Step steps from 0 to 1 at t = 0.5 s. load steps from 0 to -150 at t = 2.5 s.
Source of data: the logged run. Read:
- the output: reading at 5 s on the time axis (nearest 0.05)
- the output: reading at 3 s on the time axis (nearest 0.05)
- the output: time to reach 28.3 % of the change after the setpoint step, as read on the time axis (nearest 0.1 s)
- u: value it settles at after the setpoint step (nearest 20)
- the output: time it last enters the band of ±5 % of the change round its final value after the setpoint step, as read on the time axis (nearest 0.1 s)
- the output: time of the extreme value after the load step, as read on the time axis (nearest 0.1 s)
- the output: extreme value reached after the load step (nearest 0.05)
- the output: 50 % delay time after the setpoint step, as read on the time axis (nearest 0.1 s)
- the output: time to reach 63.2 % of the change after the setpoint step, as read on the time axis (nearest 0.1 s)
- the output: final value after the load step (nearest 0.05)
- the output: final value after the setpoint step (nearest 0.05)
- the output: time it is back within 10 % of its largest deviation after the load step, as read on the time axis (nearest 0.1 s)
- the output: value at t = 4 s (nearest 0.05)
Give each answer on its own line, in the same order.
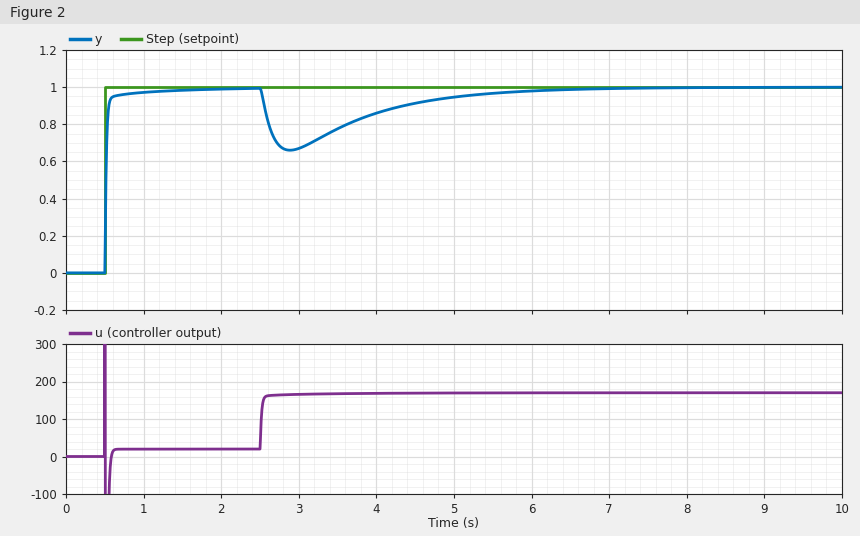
0.95
0.65
0.5 s
20
0.6 s
2.9 s
0.65
0.5 s
0.5 s
1.00
1.00
5.5 s
0.85
